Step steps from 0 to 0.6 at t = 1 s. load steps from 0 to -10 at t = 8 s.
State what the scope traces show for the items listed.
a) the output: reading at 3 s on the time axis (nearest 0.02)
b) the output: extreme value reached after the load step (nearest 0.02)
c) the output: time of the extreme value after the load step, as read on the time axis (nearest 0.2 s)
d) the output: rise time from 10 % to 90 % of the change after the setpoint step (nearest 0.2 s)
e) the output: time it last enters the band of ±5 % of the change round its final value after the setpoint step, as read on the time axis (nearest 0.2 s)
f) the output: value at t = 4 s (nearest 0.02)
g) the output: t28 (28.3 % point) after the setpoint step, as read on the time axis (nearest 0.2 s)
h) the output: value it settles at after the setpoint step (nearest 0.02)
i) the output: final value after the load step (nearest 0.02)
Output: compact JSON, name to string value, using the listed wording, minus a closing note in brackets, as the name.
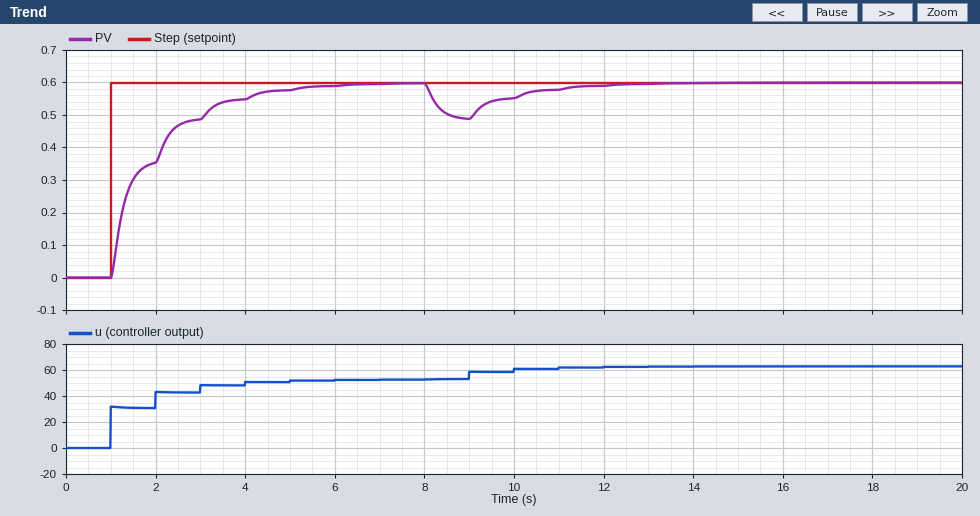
{"the output: reading at 3 s on the time axis": "0.48", "the output: extreme value reached after the load step": "0.48", "the output: time of the extreme value after the load step, as read on the time axis": "9.0 s", "the output: rise time from 10 % to 90 % of the change after the setpoint step": "2.4 s", "the output: time it last enters the band of ±5 % of the change round its final value after the setpoint step, as read on the time axis": "4.4 s", "the output: value at t = 4 s": "0.54", "the output: t28 (28.3 % point) after the setpoint step, as read on the time axis": "1.2 s", "the output: value it settles at after the setpoint step": "0.60", "the output: final value after the load step": "0.60"}
